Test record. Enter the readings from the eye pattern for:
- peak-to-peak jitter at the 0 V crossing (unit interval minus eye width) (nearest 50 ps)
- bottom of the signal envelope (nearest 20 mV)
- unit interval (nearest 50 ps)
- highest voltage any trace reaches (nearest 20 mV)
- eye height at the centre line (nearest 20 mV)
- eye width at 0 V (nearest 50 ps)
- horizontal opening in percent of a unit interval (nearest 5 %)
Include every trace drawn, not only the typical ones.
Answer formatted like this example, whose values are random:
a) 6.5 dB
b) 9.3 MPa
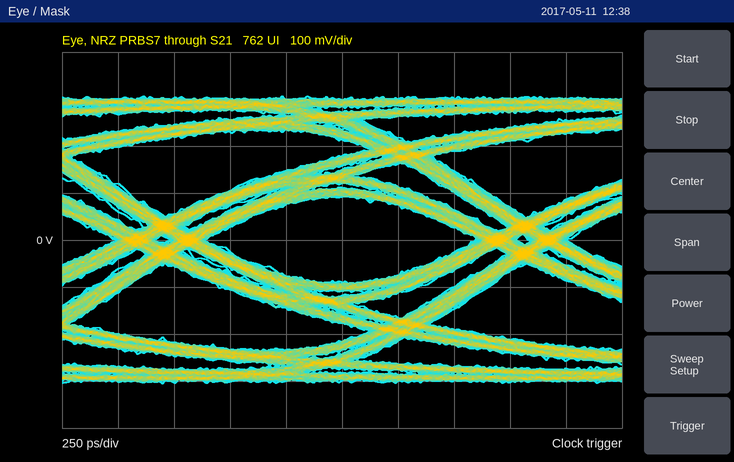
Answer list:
a) 400 ps
b) -300 mV
c) 1.60 ns
d) 300 mV
e) 180 mV
f) 1.20 ns
g) 75 %
